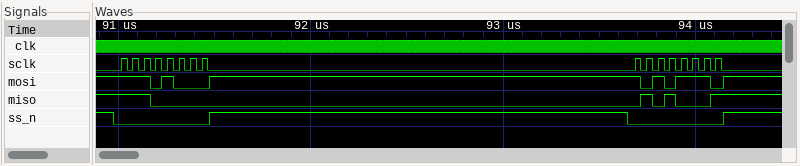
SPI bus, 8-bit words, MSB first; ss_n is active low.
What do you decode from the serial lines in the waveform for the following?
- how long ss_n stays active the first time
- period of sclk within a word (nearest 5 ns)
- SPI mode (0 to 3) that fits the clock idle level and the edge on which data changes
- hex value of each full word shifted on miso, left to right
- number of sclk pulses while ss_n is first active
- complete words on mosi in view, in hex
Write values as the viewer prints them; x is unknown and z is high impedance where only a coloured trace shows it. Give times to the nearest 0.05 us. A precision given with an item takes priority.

0.5 us
60 ns
0
E0, 51
8
E8, AE
